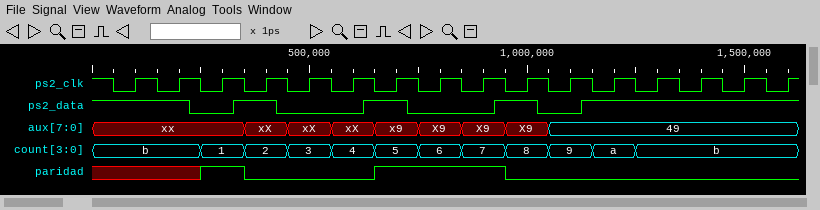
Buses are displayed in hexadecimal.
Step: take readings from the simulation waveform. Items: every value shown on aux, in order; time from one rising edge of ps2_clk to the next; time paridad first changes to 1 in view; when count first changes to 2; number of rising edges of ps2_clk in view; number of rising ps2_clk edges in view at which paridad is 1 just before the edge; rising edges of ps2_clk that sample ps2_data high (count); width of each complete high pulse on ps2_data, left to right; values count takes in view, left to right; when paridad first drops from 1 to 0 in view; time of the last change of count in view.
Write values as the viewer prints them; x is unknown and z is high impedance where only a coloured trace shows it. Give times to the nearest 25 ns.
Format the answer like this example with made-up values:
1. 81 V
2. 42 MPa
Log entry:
1. xx, xX, xX, xX, x9, X9, X9, X9, 49
2. 100 ns
3. 250 ns
4. 350 ns
5. 16
6. 4
7. 10
8. 100 ns, 100 ns, 100 ns
9. b, 1, 2, 3, 4, 5, 6, 7, 8, 9, a, b
10. 350 ns
11. 1250 ns
